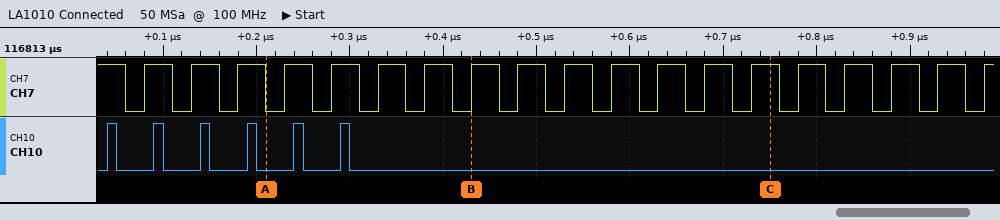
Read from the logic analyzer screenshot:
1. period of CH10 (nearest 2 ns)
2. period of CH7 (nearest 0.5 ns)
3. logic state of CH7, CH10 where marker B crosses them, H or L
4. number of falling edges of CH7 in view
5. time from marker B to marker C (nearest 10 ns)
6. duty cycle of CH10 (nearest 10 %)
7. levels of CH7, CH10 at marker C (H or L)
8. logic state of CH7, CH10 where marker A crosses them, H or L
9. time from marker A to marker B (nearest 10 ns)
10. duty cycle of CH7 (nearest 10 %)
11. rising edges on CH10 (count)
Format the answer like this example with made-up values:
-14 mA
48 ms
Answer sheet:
50 ns
50 ns
CH7=H, CH10=L
19
320 ns
20 %
CH7=H, CH10=L
CH7=L, CH10=L
220 ns
60 %
6
